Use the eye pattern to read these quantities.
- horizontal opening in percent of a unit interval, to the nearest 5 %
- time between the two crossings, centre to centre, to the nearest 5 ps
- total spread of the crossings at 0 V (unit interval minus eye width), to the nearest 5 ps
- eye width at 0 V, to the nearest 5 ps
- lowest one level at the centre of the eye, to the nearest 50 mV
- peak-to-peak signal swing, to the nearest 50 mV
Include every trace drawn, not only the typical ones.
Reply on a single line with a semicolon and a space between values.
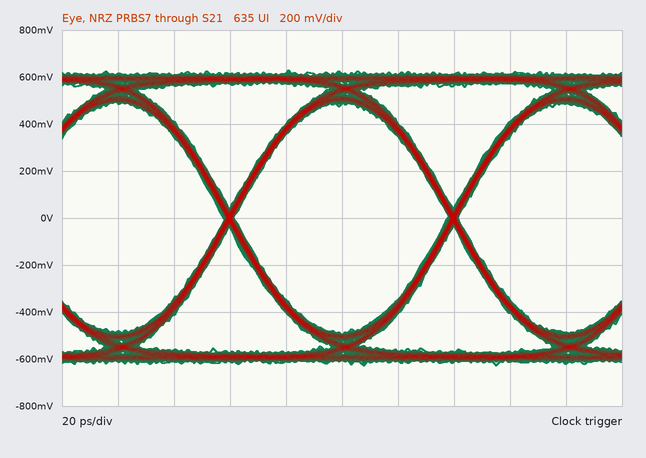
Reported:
95 %; 80 ps; 5 ps; 75 ps; 500 mV; 1.25 V
